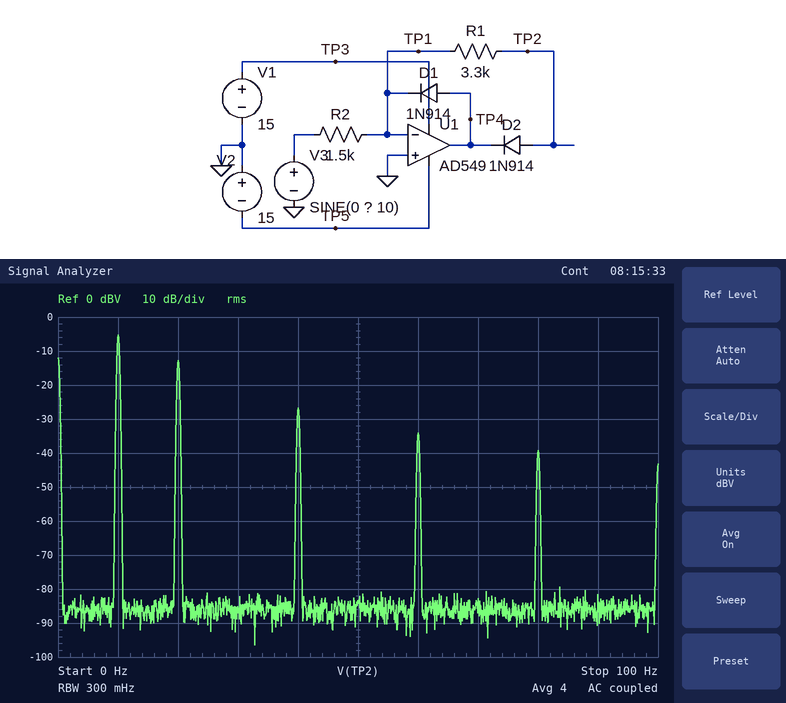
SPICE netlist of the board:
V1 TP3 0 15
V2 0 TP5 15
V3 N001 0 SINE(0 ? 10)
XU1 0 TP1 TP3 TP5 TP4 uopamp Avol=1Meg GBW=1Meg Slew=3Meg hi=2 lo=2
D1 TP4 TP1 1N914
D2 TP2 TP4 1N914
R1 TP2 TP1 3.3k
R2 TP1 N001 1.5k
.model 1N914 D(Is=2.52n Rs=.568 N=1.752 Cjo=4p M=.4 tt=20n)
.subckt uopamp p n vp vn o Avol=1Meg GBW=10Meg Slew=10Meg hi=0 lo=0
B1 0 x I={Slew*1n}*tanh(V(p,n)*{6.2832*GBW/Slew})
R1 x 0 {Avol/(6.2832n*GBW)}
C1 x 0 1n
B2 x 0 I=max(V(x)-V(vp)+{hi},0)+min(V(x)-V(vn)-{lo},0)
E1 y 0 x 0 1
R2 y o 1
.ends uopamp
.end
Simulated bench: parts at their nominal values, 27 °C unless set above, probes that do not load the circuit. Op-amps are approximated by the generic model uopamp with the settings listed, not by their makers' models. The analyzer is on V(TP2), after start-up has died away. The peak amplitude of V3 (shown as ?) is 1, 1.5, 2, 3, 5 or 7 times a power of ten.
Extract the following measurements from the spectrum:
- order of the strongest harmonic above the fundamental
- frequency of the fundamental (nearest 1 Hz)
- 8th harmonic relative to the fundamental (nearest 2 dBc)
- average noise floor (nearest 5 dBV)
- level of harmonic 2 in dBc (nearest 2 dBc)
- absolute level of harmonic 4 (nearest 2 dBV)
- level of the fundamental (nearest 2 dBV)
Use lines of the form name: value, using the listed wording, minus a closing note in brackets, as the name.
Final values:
order of the strongest harmonic above the fundamental: 2
frequency of the fundamental: 10 Hz
8th harmonic relative to the fundamental: -34 dBc
average noise floor: -85 dBV
level of harmonic 2 in dBc: -8 dBc
absolute level of harmonic 4: -26 dBV
level of the fundamental: -6 dBV
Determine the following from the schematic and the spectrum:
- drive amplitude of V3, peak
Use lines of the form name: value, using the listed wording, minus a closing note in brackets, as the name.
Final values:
drive amplitude of V3, peak: 700 mV
